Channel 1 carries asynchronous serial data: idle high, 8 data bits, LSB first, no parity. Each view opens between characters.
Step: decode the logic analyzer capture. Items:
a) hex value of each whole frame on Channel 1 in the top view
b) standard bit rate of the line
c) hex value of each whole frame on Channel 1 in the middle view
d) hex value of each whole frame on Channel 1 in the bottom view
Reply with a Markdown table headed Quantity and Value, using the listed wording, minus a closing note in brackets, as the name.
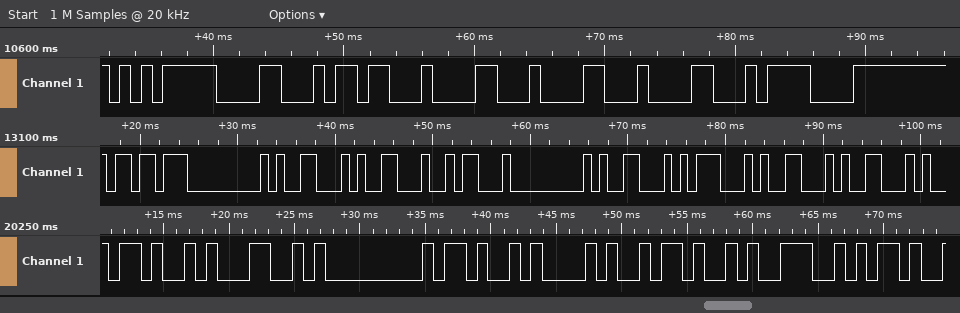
| Quantity | Value |
|---|---|
| hex value of each whole frame on Channel 1 in the top view | F5, 18, 1B, 18, 18, 18, 0F |
| standard bit rate of the line | 1200 baud |
| hex value of each whole frame on Channel 1 in the middle view | DB, 00, 19, 19, 1A, 00, 19, 1D, 19, 19 |
| hex value of each whole frame on Channel 1 in the bottom view | 4B, 4C, 00, 4B, 28, 4B, 4E |
